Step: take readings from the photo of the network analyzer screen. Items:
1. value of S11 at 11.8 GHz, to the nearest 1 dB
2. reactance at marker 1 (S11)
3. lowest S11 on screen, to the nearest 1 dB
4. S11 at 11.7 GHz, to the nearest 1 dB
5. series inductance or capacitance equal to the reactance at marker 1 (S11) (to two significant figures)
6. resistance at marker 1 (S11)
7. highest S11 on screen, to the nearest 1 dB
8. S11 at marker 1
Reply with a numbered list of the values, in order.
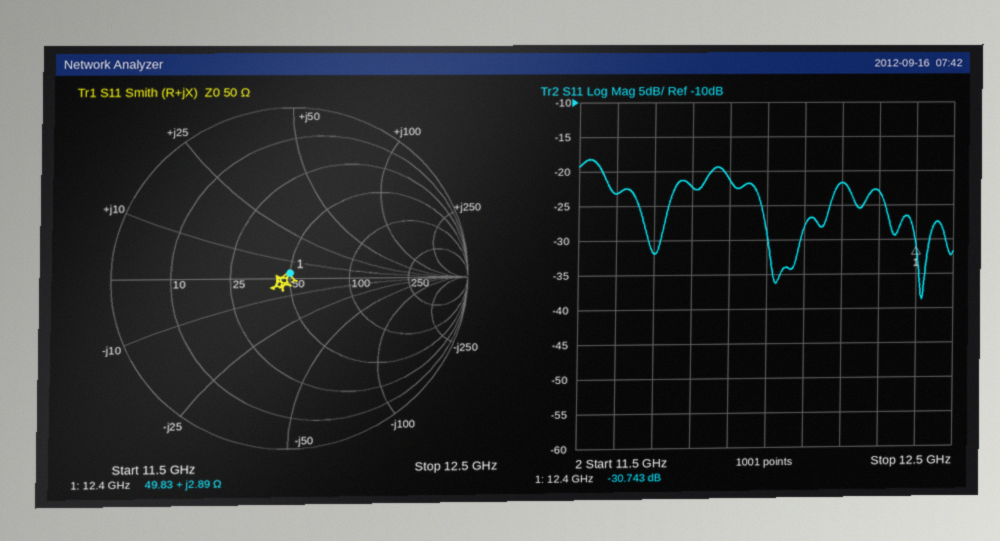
1. -22 dB
2. +2.89 Ω
3. -39 dB
4. -32 dB
5. 37 pH
6. 49.83 Ω
7. -18 dB
8. -30.743 dB
